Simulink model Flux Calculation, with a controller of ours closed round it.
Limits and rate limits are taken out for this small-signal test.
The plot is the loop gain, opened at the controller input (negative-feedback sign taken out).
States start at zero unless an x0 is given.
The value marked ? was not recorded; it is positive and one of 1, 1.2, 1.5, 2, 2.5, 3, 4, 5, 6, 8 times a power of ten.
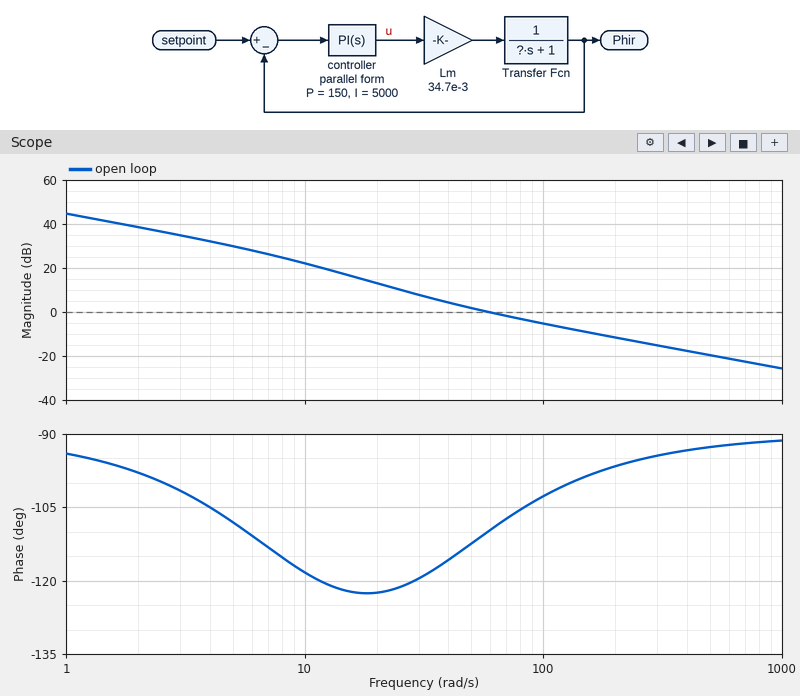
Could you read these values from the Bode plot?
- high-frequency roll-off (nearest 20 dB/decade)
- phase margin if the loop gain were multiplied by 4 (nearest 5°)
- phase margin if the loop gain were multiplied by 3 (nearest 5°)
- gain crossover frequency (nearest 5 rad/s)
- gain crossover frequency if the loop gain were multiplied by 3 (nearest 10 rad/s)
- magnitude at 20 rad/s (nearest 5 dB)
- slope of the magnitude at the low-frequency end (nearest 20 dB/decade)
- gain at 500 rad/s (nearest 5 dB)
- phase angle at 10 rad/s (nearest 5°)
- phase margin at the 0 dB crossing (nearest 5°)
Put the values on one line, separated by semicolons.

-20 dB/decade; 85°; 80°; 60 rad/s; 160 rad/s; 15 dB; -20 dB/decade; -20 dB; -120°; 70°
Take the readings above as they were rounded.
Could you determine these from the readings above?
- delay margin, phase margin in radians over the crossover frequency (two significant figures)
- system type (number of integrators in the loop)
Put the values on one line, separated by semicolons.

0.020 s; 1
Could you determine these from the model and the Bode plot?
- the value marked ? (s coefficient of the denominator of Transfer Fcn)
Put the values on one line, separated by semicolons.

0.1
